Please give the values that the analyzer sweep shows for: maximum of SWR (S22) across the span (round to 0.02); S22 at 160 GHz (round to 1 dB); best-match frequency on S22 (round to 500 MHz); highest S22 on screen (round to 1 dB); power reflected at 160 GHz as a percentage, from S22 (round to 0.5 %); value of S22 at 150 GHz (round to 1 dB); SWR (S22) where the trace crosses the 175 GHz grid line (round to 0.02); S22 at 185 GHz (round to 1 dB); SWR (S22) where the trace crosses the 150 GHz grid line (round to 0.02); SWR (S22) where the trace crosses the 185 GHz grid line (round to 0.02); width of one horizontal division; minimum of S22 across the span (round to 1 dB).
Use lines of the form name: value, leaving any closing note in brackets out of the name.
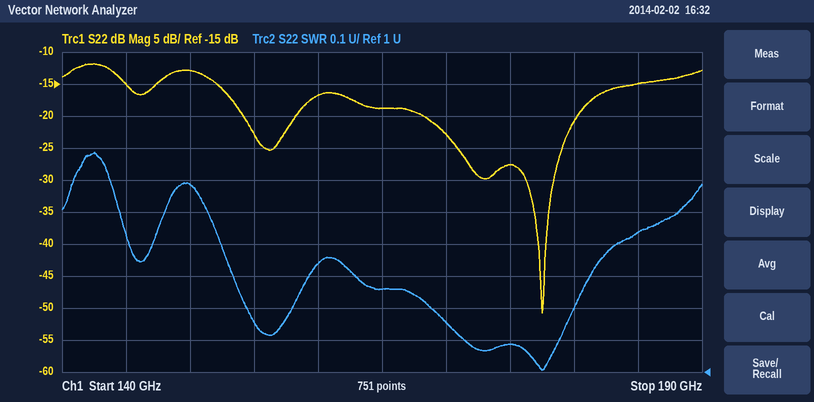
maximum of SWR (S22) across the span: 1.68
S22 at 160 GHz: -17 dB
best-match frequency on S22: 177.5 GHz
highest S22 on screen: -12 dB
power reflected at 160 GHz as a percentage, from S22: 2.0 %
value of S22 at 150 GHz: -13 dB
SWR (S22) where the trace crosses the 175 GHz grid line: 1.08
S22 at 185 GHz: -15 dB
SWR (S22) where the trace crosses the 150 GHz grid line: 1.58
SWR (S22) where the trace crosses the 185 GHz grid line: 1.44
width of one horizontal division: 5 GHz
minimum of S22 across the span: -51 dB
